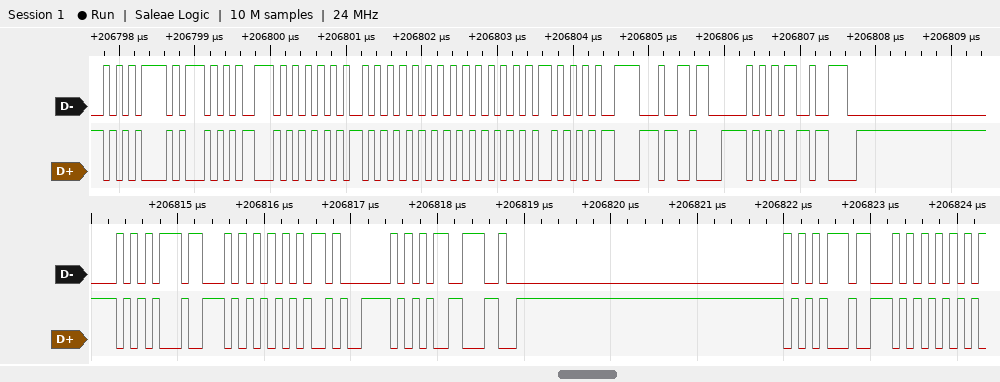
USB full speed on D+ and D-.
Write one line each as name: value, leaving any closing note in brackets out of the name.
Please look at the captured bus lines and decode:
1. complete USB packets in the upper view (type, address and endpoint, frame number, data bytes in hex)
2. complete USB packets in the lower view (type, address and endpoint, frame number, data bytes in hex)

complete USB packets in the upper view: DATA0 [ 80 06 00 01 00 00 40 00 ], ACK
complete USB packets in the lower view: IN ADDR 0 EP 0, NAK
